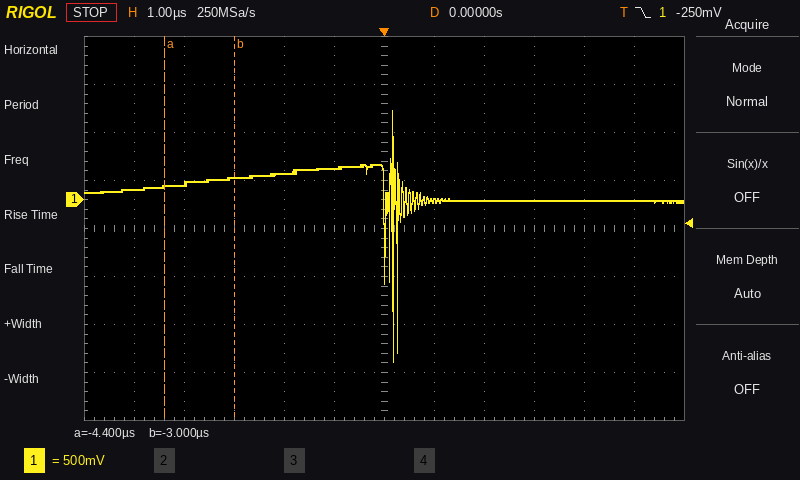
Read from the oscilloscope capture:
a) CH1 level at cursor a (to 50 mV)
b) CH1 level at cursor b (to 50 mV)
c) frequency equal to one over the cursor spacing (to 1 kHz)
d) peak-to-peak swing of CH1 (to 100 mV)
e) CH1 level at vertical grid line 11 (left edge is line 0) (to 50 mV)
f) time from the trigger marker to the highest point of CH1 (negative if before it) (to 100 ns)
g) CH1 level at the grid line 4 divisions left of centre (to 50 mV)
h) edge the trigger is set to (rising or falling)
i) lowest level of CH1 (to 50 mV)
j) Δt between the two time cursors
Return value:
150 mV
250 mV
714 kHz
2.60 V
0 mV
+200 ns
150 mV
falling
-1.70 V
1.4 µs
